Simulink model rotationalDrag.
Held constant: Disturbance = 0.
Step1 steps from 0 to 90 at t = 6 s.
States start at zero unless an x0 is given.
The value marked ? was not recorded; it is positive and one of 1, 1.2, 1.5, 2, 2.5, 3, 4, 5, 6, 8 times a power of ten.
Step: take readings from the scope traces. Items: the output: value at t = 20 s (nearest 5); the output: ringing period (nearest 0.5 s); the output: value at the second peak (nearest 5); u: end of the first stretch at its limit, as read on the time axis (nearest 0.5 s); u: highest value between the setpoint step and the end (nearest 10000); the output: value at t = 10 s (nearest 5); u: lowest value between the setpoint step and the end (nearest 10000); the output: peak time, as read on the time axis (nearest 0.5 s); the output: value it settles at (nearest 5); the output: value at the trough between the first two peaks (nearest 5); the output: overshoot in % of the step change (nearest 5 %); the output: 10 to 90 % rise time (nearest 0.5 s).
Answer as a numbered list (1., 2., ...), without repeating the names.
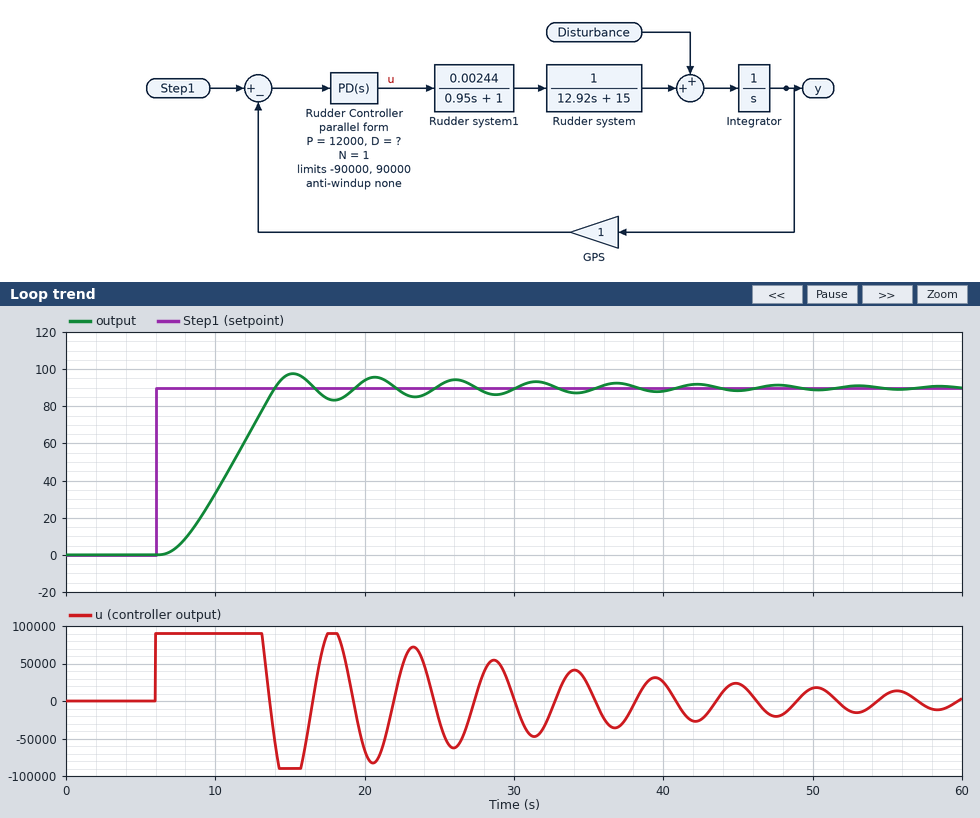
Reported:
1. 95
2. 5.5 s
3. 95
4. 13.0 s
5. 90000
6. 35
7. -90000
8. 15.0 s
9. 90
10. 85
11. 10 %
12. 5.5 s
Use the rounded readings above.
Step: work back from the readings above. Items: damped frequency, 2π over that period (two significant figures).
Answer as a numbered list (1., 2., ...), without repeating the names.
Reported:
1. 1.1 rad/s
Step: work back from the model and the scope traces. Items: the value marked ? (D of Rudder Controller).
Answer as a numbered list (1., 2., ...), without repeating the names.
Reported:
1. 4000
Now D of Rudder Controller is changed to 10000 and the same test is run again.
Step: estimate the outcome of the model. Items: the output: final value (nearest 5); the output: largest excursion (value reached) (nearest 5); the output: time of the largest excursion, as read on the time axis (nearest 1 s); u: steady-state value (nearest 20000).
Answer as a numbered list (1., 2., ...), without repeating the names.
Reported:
1. 90
2. 95
3. 19 s
4. 0
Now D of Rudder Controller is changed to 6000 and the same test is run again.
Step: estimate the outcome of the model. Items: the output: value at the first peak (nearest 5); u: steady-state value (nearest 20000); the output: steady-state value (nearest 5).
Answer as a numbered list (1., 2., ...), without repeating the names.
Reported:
1. 95
2. 0
3. 90
